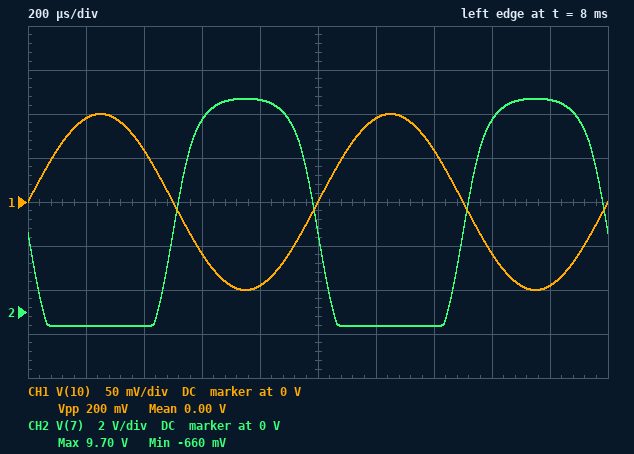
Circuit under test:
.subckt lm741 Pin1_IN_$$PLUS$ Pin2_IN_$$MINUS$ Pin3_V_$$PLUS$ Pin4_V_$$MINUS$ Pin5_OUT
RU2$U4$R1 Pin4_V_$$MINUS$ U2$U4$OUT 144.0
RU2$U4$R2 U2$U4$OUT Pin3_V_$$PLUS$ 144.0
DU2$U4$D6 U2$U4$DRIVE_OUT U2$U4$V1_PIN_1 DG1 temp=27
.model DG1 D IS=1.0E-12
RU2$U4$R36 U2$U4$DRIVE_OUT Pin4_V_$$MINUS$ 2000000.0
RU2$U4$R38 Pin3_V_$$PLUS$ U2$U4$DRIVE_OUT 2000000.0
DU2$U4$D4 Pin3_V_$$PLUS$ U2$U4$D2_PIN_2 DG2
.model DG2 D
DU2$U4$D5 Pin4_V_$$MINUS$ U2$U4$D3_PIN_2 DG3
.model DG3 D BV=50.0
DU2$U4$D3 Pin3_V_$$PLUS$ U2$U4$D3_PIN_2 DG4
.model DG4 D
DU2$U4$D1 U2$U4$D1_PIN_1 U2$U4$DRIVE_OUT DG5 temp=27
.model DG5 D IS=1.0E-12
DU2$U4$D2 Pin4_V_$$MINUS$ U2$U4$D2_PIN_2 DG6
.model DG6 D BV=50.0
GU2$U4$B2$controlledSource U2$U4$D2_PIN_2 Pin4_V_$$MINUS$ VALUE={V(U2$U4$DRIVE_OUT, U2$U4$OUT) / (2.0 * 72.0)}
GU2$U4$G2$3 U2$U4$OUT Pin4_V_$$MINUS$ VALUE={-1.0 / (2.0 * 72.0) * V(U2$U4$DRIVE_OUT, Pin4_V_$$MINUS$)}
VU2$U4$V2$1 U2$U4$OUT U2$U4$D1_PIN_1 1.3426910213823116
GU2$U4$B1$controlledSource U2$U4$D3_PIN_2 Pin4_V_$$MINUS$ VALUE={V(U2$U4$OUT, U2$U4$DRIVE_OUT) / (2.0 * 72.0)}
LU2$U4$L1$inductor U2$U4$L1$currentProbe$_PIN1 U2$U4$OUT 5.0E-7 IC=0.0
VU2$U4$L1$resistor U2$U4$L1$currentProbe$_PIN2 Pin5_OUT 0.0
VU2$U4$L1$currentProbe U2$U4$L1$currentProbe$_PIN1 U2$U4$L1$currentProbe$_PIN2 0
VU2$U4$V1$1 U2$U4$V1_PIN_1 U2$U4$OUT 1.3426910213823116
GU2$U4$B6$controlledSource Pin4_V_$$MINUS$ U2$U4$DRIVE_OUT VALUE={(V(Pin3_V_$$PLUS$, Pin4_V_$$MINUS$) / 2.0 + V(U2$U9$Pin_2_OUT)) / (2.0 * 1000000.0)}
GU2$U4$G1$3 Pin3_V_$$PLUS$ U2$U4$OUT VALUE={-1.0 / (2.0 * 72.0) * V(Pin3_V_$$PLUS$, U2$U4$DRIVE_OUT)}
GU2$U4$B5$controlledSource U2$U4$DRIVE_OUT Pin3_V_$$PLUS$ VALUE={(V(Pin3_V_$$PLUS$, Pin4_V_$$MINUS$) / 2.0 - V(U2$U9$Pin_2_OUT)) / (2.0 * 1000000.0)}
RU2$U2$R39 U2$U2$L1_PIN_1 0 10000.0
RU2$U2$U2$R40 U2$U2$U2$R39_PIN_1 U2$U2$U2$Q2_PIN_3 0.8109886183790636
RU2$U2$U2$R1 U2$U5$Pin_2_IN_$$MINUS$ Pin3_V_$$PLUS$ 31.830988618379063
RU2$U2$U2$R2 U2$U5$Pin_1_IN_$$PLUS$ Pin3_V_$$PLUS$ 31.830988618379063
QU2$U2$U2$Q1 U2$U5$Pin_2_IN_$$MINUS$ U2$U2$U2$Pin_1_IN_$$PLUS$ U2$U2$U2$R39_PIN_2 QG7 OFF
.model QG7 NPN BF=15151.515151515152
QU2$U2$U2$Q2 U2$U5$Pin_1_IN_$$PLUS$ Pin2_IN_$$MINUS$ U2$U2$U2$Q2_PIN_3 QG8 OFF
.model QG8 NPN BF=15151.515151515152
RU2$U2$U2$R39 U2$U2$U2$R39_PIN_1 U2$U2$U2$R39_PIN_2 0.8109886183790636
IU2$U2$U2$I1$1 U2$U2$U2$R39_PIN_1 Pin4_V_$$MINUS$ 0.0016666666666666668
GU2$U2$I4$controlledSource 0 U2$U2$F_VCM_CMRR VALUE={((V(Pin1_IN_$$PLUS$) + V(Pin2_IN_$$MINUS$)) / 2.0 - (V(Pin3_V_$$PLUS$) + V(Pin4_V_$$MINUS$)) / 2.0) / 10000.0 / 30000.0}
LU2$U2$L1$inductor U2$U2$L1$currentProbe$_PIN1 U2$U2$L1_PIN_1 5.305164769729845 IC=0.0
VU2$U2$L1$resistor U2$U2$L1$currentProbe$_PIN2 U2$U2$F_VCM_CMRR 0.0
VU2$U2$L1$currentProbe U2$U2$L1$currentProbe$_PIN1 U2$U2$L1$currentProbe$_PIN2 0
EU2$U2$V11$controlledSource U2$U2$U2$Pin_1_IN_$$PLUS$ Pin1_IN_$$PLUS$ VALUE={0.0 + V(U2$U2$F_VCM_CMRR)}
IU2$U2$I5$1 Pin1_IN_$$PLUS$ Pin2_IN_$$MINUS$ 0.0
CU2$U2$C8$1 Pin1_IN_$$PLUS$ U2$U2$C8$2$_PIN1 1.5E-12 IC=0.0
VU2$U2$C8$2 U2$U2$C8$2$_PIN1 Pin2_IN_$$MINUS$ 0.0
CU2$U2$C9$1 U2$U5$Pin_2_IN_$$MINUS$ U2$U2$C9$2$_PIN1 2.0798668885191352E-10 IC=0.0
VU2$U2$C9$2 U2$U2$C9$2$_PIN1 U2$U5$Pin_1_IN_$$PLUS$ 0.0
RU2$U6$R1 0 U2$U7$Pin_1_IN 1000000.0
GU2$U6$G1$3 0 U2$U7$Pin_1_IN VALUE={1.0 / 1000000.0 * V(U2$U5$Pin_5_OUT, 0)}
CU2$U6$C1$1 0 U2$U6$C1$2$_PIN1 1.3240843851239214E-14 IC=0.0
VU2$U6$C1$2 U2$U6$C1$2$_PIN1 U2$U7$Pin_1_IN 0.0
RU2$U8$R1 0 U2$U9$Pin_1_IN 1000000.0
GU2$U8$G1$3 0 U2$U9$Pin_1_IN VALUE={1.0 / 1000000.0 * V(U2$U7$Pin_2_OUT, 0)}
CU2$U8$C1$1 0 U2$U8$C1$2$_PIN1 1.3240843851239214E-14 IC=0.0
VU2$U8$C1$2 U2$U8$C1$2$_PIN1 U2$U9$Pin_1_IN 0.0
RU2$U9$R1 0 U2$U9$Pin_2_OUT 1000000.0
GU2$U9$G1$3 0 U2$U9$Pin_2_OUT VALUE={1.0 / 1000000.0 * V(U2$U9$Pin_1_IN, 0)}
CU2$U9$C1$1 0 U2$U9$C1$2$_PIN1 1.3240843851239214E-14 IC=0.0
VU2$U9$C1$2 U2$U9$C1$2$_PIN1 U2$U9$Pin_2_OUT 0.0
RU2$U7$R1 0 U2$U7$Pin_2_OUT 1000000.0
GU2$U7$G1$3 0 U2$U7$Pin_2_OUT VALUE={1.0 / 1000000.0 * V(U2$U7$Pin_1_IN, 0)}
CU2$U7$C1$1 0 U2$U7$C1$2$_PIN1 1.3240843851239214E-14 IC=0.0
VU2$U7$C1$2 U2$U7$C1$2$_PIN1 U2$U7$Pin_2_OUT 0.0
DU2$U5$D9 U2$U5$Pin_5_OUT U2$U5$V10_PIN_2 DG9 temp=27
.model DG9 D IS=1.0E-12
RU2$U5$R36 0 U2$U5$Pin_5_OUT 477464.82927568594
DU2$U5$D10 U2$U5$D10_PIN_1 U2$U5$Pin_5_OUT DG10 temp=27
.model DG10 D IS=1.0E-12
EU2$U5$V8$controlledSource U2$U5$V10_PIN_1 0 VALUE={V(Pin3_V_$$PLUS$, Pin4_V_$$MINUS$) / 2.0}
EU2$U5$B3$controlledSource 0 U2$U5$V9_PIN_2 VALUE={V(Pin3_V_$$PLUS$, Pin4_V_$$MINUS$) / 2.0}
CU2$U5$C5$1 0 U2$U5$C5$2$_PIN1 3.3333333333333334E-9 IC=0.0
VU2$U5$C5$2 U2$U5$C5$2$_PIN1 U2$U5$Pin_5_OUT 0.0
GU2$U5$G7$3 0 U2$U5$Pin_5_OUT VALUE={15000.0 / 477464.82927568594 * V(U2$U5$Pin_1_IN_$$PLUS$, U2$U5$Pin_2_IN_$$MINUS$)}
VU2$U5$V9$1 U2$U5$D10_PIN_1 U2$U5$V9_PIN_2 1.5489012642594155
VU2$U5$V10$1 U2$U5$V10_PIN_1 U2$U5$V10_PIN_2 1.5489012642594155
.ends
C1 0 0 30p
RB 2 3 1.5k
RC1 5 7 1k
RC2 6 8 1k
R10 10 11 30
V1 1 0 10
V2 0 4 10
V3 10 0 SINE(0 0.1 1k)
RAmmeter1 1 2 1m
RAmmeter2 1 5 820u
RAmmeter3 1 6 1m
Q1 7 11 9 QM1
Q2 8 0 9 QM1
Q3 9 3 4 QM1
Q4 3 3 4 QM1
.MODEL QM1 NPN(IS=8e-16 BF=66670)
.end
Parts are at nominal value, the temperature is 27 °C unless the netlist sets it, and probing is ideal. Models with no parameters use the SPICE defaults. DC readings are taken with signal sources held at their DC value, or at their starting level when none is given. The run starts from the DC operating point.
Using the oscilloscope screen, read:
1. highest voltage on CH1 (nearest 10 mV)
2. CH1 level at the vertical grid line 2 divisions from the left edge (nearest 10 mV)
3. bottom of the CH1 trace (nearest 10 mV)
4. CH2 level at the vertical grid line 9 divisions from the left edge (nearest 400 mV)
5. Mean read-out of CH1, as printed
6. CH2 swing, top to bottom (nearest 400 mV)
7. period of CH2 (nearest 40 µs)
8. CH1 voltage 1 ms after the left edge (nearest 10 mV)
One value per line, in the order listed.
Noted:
100 mV
60 mV
-100 mV
9.6 V
0.00 V
10.4 V
1.00 ms
0 V
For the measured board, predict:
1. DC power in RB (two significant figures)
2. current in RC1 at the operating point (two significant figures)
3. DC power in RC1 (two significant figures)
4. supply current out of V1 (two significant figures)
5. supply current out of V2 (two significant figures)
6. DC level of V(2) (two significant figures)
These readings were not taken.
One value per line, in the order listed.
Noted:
250 mW
6.4 mA
41 mW
26 mA
26 mA
10 V
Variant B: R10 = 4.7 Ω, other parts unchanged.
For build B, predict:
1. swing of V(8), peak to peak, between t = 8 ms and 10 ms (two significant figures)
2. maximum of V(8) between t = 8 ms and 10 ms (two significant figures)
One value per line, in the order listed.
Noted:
10 V
9.6 V
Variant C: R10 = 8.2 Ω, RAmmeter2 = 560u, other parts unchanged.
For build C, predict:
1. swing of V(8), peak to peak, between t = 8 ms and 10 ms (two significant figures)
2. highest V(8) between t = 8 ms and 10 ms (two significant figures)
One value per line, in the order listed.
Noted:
10 V
9.5 V
